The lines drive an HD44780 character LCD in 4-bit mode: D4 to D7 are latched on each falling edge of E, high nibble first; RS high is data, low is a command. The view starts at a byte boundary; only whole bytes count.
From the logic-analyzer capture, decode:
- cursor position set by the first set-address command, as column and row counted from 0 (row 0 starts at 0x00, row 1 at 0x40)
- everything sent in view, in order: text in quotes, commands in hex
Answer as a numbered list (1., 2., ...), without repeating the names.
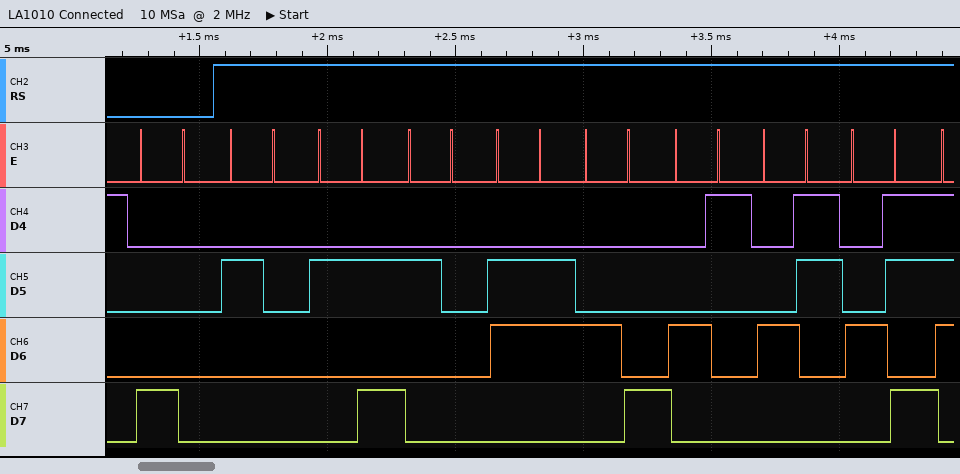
1. column 0, row 0
2. 0x80 " * fHACK"
